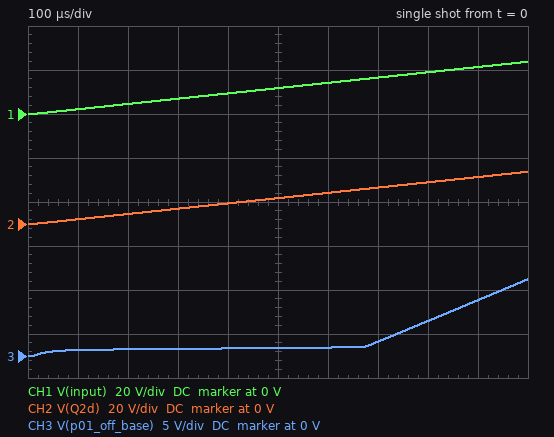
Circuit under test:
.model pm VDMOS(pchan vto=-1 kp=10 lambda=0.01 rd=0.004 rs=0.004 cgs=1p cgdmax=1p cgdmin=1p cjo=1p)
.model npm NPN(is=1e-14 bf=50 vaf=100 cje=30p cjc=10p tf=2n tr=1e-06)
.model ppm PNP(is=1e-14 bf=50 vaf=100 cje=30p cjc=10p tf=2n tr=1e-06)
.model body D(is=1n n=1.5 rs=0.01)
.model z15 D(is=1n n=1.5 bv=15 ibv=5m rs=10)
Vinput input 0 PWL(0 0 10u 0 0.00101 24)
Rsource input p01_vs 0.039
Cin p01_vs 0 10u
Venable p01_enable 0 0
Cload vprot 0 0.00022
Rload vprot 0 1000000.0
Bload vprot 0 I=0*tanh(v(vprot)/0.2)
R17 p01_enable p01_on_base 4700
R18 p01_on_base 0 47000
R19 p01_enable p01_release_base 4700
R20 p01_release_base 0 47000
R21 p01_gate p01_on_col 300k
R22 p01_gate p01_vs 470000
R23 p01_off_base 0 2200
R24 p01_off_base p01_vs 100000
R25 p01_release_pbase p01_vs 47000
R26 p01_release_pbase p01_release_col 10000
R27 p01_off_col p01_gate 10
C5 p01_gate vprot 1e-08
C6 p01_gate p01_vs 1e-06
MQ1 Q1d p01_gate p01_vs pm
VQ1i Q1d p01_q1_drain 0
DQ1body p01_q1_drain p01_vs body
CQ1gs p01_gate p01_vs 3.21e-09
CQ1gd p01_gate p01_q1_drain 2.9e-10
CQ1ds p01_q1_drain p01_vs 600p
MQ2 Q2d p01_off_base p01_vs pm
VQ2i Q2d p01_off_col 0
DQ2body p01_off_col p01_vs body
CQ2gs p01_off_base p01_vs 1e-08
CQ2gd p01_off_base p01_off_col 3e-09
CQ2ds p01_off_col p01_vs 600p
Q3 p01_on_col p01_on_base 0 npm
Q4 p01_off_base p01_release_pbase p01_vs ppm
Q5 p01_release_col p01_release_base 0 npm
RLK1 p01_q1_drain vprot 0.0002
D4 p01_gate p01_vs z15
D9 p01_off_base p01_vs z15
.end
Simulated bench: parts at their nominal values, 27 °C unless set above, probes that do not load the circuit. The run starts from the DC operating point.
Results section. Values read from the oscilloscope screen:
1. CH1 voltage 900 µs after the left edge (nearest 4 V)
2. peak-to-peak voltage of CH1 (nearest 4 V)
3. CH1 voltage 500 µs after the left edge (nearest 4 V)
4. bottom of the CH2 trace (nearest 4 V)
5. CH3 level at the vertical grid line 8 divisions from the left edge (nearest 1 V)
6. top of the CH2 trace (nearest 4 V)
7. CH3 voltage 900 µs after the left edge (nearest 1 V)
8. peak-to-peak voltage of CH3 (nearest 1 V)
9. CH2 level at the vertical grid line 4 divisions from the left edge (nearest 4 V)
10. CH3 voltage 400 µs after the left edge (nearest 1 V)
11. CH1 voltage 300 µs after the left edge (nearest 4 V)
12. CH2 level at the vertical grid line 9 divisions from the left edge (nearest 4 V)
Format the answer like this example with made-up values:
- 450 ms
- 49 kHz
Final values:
- 20 V
- 24 V
- 12 V
- 0 V
- 4 V
- 24 V
- 6 V
- 9 V
- 8 V
- 1 V
- 8 V
- 20 V
